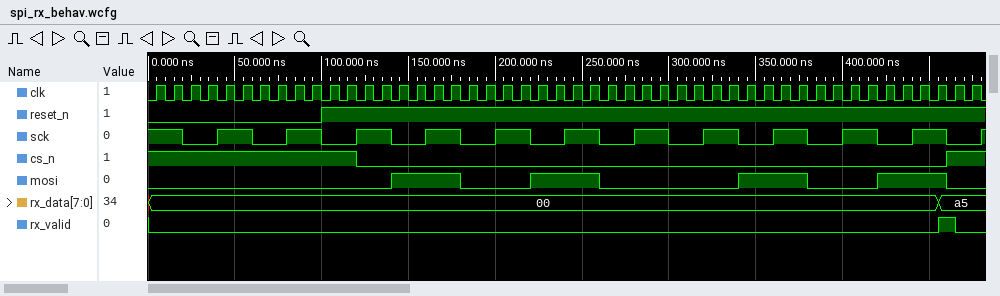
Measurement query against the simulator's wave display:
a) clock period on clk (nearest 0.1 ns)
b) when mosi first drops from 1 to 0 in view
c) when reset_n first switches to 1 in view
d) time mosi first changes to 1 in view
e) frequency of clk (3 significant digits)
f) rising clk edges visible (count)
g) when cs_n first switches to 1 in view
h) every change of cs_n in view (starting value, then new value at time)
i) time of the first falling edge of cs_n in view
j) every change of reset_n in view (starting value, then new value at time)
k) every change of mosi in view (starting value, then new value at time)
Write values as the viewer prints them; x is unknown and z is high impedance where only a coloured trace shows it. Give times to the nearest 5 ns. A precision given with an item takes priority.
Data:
10 ns
180 ns
100 ns
140 ns
100 MHz
48
460 ns
1, 0 at 120 ns, 1 at 460 ns
120 ns
0, 1 at 100 ns
0, 1 at 140 ns, 0 at 180 ns, 1 at 220 ns, 0 at 260 ns, 1 at 340 ns, 0 at 380 ns, 1 at 420 ns, 0 at 460 ns
